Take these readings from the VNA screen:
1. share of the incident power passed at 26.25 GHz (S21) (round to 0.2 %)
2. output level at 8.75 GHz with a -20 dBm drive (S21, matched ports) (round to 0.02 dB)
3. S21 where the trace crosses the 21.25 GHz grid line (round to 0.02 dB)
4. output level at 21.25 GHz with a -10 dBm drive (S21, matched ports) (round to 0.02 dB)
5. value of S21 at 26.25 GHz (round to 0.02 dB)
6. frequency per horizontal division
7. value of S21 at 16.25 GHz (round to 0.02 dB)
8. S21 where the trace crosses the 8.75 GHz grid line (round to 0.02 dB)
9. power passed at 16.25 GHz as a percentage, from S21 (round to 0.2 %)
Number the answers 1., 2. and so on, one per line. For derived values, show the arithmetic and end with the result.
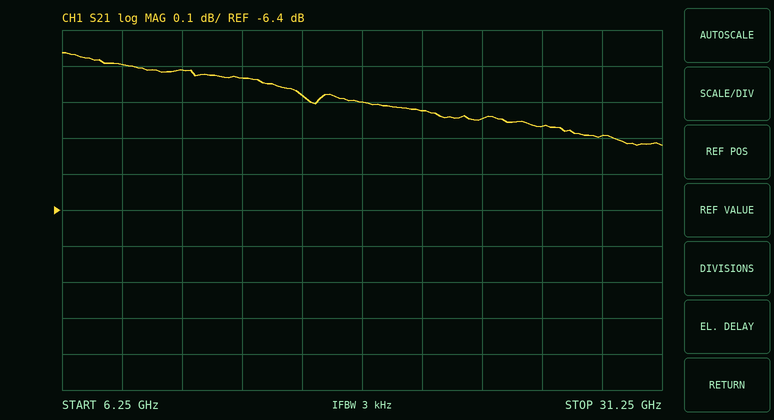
1. 10^(-6.16/10) ≈ 24.2 %
2. -20 dBm + (-6.00 dB) = -26.00 dBm
3. -6.12 dB
4. -10 dBm + (-6.12 dB) = -16.12 dBm
5. -6.16 dB
6. 2.5 GHz
7. -6.08 dB
8. -6.00 dB
9. 10^(-6.08/10) ≈ 24.7 %, so 24.6 % to the nearest 0.2 %
